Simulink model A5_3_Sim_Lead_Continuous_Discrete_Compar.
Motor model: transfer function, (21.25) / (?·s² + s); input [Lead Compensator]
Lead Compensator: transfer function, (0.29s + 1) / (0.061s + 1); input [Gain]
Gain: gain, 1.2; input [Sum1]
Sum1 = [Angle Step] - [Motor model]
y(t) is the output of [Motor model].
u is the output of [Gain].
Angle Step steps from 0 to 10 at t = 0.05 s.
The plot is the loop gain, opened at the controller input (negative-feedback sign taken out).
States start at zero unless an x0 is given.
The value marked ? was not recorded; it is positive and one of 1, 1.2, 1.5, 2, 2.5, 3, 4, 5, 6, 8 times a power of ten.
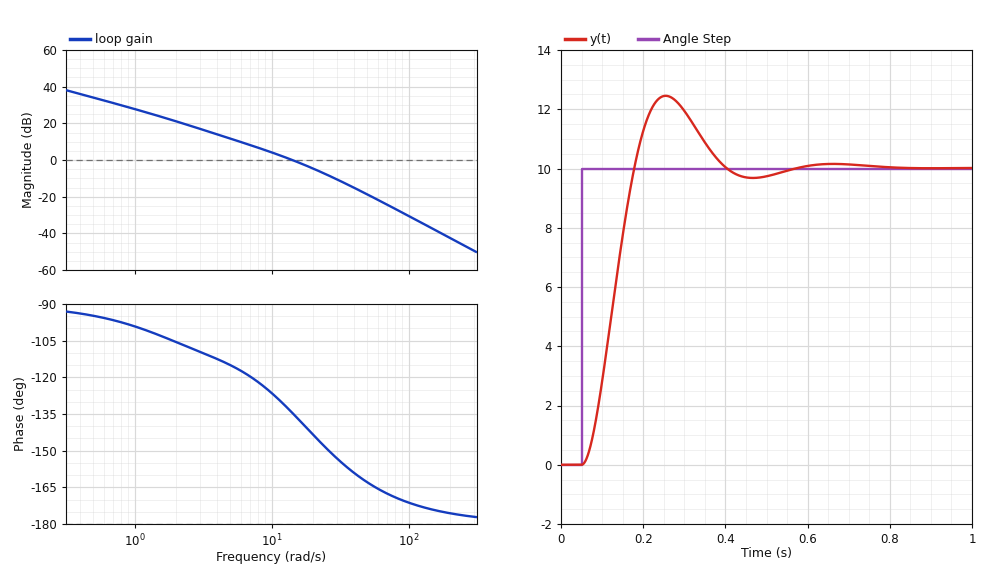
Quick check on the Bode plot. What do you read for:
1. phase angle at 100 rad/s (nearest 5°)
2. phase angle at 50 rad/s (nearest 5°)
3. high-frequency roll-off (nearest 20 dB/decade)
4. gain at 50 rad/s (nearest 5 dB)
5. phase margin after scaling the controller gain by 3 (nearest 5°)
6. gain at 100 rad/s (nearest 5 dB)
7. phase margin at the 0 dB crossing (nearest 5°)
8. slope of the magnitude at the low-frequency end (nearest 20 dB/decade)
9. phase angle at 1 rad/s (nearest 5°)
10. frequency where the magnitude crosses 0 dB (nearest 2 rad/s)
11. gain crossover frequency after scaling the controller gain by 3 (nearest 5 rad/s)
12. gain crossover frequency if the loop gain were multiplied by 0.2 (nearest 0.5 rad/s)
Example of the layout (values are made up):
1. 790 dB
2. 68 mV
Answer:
1. -170°
2. -165°
3. -40 dB/decade
4. -20 dB
5. 30°
6. -30 dB
7. 45°
8. -20 dB/decade
9. -100°
10. 14 rad/s
11. 30 rad/s
12. 4.0 rad/s
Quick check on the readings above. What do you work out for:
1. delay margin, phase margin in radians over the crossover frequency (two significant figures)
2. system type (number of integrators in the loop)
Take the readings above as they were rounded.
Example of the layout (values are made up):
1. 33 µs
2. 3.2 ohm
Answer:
1. 0.056 s
2. 1
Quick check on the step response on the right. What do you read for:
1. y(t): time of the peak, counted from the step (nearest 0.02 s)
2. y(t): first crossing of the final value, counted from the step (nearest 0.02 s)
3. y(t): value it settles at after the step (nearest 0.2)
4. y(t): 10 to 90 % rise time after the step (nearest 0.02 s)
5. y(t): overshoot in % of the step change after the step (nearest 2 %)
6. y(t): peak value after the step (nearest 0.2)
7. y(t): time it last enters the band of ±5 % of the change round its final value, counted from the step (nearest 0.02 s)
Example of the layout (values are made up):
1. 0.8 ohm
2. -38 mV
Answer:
1. 0.20 s
2. 0.12 s
3. 10.0
4. 0.08 s
5. 24 %
6. 12.4
7. 0.32 s
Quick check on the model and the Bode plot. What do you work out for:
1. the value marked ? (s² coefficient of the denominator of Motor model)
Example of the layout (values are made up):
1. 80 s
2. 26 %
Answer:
1. 0.4
